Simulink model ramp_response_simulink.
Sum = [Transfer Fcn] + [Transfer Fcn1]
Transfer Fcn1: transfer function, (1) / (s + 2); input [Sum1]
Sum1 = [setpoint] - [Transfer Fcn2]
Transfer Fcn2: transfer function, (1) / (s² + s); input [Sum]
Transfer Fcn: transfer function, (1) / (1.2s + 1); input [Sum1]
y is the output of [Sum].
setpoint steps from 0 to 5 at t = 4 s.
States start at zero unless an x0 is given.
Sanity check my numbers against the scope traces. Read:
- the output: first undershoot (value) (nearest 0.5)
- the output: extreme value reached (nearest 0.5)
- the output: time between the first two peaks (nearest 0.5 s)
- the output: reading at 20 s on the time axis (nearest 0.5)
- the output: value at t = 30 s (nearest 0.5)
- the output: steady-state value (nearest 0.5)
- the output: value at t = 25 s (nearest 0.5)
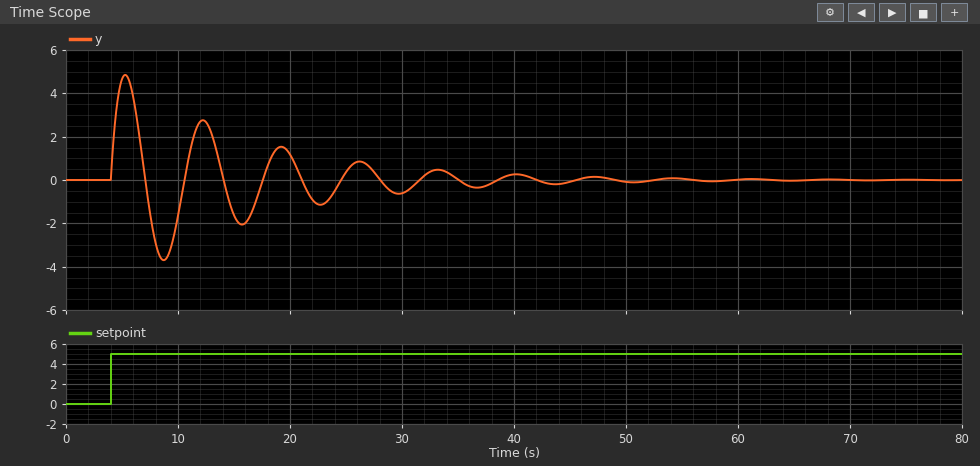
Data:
-3.5
5.0
7.0 s
1.0
-0.5
0.0
0.5
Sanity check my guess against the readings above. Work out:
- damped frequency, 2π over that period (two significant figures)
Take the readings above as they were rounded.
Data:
0.90 rad/s
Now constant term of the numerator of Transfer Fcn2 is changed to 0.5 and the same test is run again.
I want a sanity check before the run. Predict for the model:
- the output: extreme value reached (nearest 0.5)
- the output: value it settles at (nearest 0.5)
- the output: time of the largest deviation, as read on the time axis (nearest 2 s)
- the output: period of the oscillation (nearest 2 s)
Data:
5.5
0.0
6 s
10 s
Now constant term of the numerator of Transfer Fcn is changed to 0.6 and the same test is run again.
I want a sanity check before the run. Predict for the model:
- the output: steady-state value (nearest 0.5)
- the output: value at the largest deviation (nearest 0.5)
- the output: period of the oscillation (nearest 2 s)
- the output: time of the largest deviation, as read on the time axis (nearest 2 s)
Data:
0.0
4.0
8 s
6 s
